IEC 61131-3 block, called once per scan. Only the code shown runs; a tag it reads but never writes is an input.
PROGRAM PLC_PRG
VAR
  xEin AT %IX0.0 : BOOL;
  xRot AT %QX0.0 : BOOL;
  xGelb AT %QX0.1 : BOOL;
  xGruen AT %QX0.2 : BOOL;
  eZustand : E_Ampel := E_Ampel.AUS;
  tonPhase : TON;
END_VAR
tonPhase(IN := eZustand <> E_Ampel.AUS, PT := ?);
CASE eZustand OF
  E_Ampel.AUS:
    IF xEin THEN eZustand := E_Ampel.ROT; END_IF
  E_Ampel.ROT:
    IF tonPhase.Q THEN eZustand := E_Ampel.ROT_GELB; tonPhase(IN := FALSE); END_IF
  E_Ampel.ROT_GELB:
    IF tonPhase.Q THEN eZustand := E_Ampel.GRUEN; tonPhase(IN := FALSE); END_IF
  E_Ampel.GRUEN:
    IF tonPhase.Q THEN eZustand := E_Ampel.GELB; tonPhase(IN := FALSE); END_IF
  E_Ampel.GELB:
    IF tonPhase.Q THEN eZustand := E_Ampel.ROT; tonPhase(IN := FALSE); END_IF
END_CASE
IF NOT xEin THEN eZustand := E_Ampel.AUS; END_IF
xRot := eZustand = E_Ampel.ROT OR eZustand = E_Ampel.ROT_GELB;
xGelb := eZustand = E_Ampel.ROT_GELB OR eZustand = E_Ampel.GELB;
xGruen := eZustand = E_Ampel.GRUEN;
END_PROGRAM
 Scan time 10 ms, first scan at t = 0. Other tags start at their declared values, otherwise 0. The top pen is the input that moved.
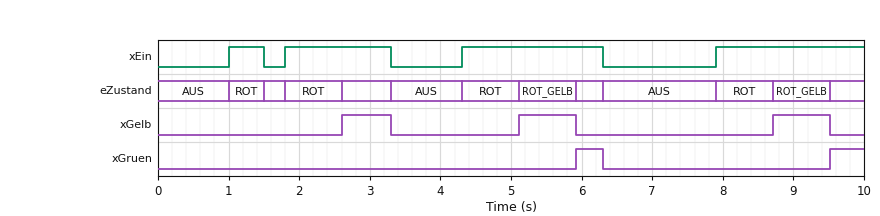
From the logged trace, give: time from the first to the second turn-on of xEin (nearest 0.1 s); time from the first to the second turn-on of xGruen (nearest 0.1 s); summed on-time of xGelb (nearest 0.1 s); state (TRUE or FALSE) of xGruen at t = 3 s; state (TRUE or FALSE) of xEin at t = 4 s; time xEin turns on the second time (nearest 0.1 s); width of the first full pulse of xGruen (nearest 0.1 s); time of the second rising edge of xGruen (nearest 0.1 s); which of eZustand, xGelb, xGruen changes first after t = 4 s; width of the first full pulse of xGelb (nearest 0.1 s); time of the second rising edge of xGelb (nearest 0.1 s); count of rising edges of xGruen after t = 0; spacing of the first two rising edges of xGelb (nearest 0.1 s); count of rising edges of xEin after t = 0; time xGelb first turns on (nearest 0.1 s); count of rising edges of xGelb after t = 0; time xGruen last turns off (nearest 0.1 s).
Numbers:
0.8 s
3.6 s
2.3 s
FALSE
FALSE
1.8 s
0.4 s
9.5 s
eZustand
0.7 s
5.1 s
2
2.5 s
4
2.6 s
3
6.3 s
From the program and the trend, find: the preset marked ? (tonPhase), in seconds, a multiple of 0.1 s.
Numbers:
0.8 s
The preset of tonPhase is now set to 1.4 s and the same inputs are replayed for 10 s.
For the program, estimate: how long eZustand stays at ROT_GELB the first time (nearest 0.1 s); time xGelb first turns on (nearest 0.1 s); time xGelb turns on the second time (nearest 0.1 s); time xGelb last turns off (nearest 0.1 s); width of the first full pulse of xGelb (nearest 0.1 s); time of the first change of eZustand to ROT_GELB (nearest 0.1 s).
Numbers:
0.1 s
3.2 s
5.7 s
6.3 s
0.1 s
3.2 s
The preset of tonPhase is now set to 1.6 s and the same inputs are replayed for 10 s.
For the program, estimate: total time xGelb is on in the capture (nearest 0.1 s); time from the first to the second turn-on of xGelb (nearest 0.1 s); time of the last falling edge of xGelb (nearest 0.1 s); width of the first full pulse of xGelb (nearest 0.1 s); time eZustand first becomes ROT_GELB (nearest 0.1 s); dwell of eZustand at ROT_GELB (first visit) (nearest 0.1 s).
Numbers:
0.9 s
3.6 s
6.3 s
0.4 s
5.9 s
0.4 s
